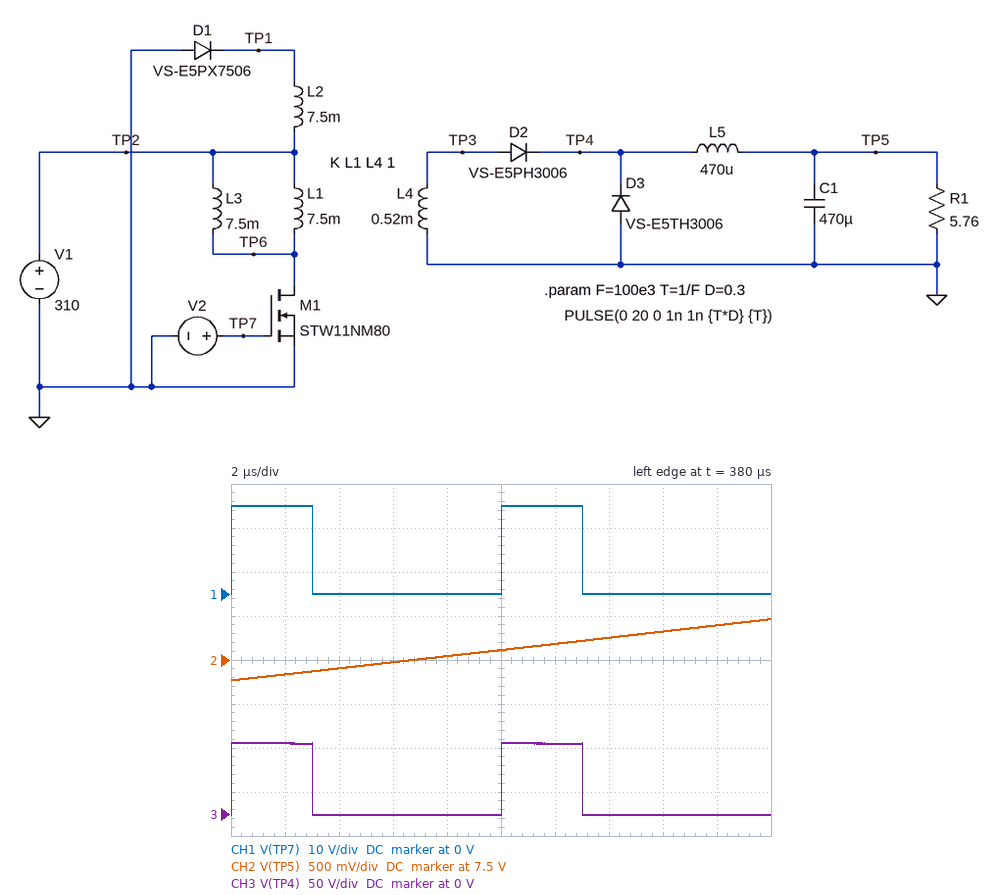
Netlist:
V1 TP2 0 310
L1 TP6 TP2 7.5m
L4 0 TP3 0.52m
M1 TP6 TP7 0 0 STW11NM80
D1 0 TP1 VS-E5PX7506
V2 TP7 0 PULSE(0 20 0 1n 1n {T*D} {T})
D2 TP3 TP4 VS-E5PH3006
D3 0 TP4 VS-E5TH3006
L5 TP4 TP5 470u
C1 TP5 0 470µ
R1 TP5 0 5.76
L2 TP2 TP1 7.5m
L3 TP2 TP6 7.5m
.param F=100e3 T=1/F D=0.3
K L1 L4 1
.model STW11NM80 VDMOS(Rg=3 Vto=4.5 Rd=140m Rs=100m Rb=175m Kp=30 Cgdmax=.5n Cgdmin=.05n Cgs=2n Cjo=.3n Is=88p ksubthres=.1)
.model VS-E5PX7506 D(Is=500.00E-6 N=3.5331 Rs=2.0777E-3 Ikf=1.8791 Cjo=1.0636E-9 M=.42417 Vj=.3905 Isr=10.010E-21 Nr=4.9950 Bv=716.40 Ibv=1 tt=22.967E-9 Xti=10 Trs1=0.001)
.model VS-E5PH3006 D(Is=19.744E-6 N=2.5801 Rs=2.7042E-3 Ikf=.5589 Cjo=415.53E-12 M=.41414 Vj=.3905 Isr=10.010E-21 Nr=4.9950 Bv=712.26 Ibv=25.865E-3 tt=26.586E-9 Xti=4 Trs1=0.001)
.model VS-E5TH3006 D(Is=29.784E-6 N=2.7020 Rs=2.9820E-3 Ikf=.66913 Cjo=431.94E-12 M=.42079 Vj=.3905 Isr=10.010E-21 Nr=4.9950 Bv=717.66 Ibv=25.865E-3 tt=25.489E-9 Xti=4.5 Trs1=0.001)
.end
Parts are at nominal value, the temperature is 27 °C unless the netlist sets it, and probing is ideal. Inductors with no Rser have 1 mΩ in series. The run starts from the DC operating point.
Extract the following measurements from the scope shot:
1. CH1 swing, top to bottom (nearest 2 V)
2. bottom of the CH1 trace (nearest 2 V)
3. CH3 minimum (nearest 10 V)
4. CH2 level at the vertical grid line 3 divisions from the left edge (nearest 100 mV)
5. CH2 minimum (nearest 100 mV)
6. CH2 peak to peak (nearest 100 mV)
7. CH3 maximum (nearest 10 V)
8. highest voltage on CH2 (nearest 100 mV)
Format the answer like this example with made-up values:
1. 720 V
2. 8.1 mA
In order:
1. 20 V
2. 0 V
3. 0 V
4. 7.5 V
5. 7.3 V
6. 700 mV
7. 80 V
8. 8.0 V
